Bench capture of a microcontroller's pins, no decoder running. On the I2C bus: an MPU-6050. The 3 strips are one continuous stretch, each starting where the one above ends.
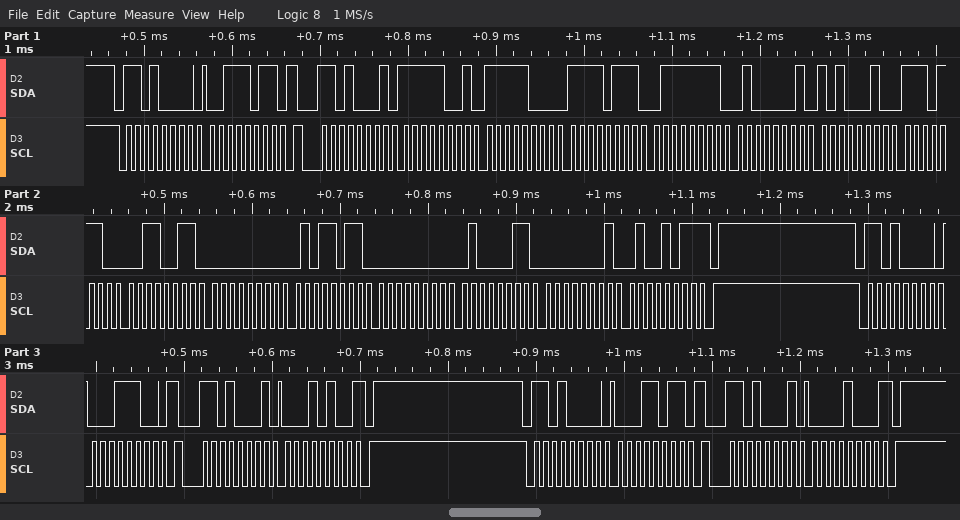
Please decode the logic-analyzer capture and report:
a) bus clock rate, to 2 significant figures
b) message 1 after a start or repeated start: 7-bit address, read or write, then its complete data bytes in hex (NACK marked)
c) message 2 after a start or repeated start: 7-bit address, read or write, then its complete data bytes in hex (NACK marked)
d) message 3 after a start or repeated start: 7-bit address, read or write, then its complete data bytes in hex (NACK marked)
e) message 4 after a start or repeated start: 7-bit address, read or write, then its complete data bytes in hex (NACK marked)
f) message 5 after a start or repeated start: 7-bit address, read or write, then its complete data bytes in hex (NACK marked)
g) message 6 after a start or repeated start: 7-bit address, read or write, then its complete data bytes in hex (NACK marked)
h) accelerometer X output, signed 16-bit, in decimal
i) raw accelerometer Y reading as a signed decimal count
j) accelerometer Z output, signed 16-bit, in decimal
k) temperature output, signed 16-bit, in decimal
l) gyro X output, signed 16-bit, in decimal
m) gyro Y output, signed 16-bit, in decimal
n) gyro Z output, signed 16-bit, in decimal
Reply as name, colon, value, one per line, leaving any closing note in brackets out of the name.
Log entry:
bus clock rate, to 2 significant figures: 100 kHz
message 1 after a start or repeated start: 7-bit address, read or write, then its complete data bytes in hex: 0x68 write: 3B
message 2 after a start or repeated start: 7-bit address, read or write, then its complete data bytes in hex: 0x68 read: F9 F8 F7 7F 41 A2 EE 33 00 5B 00 43 01 4B NACK
message 3 after a start or repeated start: 7-bit address, read or write, then its complete data bytes in hex: 0x68 write: 1C
message 4 after a start or repeated start: 7-bit address, read or write, then its complete data bytes in hex: 0x68 read: 14 NACK
message 5 after a start or repeated start: 7-bit address, read or write, then its complete data bytes in hex: 0x68 write: 1B
message 6 after a start or repeated start: 7-bit address, read or write, then its complete data bytes in hex: 0x68 read: 08 NACK
accelerometer X output, signed 16-bit, in decimal: -1544
raw accelerometer Y reading as a signed decimal count: -2177
accelerometer Z output, signed 16-bit, in decimal: 16802
temperature output, signed 16-bit, in decimal: -4557
gyro X output, signed 16-bit, in decimal: 91
gyro Y output, signed 16-bit, in decimal: 67
gyro Z output, signed 16-bit, in decimal: 331
